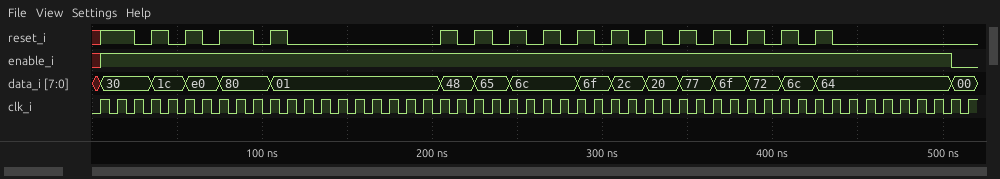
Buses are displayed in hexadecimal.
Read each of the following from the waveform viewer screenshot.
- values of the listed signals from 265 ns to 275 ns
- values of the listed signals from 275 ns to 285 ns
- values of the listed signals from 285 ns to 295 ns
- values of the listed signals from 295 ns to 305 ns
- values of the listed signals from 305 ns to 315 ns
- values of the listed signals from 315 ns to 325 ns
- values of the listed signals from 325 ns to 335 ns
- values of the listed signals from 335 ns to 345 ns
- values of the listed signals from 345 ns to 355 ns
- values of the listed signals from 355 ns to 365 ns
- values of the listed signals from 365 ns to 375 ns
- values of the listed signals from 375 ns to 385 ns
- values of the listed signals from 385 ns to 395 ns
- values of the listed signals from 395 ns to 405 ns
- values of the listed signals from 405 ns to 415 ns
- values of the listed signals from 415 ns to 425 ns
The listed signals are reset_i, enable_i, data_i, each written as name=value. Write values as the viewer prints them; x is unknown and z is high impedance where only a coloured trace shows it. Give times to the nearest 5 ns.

reset_i=1, enable_i=1, data_i=6c
reset_i=0, enable_i=1, data_i=6c
reset_i=1, enable_i=1, data_i=6f
reset_i=0, enable_i=1, data_i=6f
reset_i=1, enable_i=1, data_i=2c
reset_i=0, enable_i=1, data_i=2c
reset_i=1, enable_i=1, data_i=20
reset_i=0, enable_i=1, data_i=20
reset_i=1, enable_i=1, data_i=77
reset_i=0, enable_i=1, data_i=77
reset_i=1, enable_i=1, data_i=6f
reset_i=0, enable_i=1, data_i=6f
reset_i=1, enable_i=1, data_i=72
reset_i=0, enable_i=1, data_i=72
reset_i=1, enable_i=1, data_i=6c
reset_i=0, enable_i=1, data_i=6c
